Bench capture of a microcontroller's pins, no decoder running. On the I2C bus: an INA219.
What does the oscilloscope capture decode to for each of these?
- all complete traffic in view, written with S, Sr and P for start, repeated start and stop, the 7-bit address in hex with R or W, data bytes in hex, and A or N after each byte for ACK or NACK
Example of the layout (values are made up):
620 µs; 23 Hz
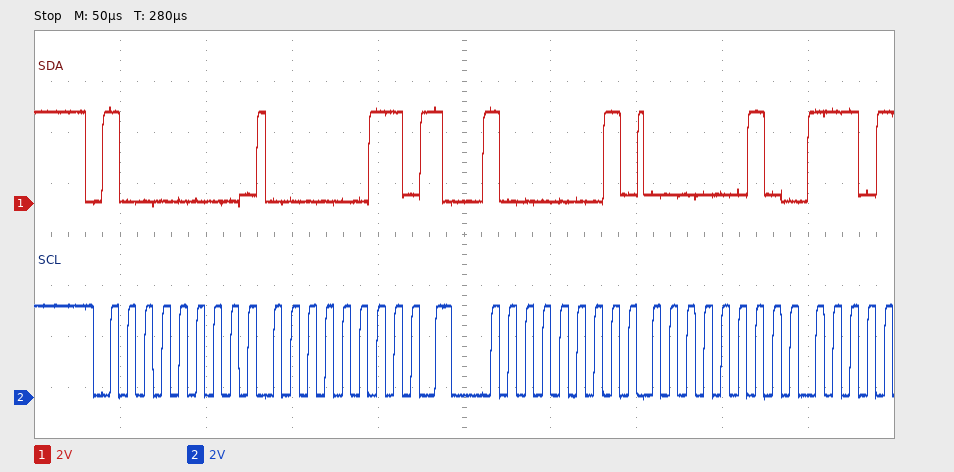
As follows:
S 40W A 03 A Sr 40R A 02 A
